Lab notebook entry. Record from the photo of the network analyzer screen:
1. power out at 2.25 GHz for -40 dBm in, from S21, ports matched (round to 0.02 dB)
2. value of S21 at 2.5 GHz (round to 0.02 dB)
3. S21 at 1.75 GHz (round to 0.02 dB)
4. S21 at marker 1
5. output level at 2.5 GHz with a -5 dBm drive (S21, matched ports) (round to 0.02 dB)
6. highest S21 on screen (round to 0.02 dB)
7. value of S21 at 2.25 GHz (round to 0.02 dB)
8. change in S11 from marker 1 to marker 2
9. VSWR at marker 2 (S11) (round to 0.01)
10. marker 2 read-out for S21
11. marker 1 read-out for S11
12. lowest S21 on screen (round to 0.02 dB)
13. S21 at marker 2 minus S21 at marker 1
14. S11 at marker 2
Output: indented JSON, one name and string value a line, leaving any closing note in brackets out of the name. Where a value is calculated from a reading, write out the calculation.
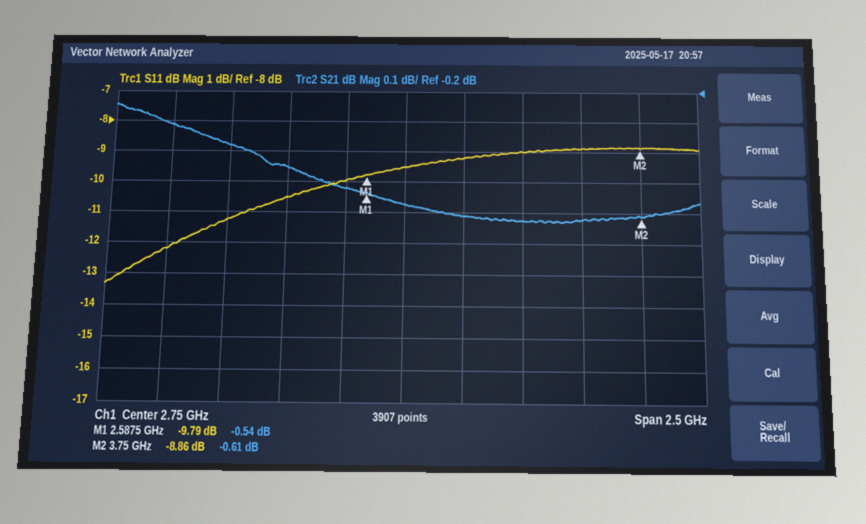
{
  "power out at 2.25 GHz for -40 dBm in, from S21, ports matched": "-40 dBm + (-0.46 dB) = -40.46 dBm",
  "value of S21 at 2.5 GHz": "-0.52 dB",
  "S21 at 1.75 GHz": "-0.32 dB",
  "S21 at marker 1": "-0.54 dB",
  "output level at 2.5 GHz with a -5 dBm drive (S21, matched ports)": "-5 dBm + (-0.52 dB) = -5.52 dBm",
  "highest S21 on screen": "-0.24 dB",
  "value of S21 at 2.25 GHz": "-0.46 dB",
  "change in S11 from marker 1 to marker 2": "-8.86 − (-9.79) = 0.93 dB",
  "VSWR at marker 2 (S11)": "(1 + 0.3606)/(1 − 0.3606) ≈ 2.13",
  "marker 2 read-out for S21": "-0.61 dB",
  "marker 1 read-out for S11": "-9.79 dB",
  "lowest S21 on screen": "-0.64 dB",
  "S21 at marker 2 minus S21 at marker 1": "-0.61 − (-0.54) = -0.07 dB",
  "S11 at marker 2": "-8.86 dB"
}
